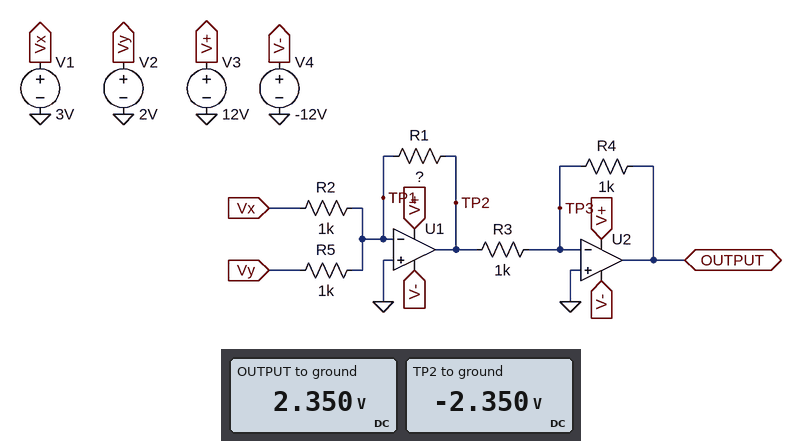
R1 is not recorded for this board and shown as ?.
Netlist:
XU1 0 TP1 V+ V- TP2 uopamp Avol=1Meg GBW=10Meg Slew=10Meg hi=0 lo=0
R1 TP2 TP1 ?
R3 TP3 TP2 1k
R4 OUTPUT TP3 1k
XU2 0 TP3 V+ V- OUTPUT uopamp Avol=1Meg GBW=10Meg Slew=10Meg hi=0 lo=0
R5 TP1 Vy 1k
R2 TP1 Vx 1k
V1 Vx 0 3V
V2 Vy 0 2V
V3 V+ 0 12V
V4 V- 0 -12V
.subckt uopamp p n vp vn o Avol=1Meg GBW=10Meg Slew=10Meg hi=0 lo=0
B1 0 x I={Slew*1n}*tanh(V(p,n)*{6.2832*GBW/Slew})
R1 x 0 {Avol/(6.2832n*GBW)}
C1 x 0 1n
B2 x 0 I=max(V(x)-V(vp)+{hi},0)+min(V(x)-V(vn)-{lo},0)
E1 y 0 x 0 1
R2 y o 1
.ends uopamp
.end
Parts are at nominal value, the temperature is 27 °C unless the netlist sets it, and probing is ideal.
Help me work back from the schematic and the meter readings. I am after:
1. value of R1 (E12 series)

470 Ω
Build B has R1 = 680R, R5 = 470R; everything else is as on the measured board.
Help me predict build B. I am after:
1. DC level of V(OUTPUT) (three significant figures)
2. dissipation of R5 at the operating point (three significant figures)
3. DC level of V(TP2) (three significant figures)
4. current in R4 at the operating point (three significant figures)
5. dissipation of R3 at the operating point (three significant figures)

4.93 V
8.51 mW
-4.93 V
4.93 mA
24.3 mW
